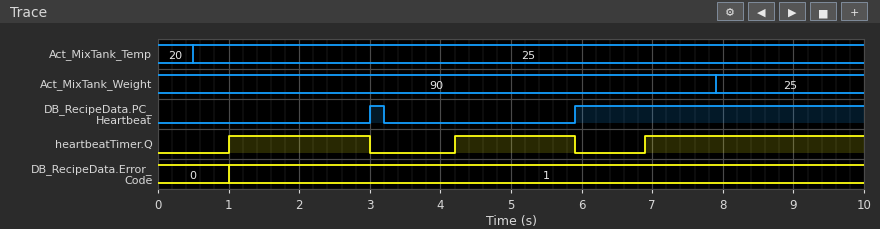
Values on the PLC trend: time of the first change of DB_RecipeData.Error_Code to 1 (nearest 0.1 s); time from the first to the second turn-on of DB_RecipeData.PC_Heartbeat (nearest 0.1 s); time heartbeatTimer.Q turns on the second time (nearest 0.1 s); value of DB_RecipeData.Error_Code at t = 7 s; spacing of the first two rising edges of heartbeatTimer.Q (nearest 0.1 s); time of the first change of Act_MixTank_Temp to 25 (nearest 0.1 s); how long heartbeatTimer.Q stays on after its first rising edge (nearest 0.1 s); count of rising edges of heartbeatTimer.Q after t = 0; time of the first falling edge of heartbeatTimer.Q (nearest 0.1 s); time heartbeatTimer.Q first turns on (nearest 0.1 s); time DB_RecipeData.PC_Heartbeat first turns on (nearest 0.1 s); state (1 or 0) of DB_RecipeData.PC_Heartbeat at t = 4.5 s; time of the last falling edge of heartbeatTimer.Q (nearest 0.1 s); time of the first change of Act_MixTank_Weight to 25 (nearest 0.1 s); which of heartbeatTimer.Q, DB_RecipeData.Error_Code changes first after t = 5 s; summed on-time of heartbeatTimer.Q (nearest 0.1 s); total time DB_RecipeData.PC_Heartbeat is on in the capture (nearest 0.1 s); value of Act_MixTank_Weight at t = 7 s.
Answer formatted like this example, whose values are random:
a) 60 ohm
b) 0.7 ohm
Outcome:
a) 1.0 s
b) 2.9 s
c) 4.2 s
d) 1
e) 3.2 s
f) 0.5 s
g) 2.0 s
h) 3
i) 3.0 s
j) 1.0 s
k) 3.0 s
l) 0
m) 5.9 s
n) 7.9 s
o) heartbeatTimer.Q
p) 6.8 s
q) 4.3 s
r) 90
